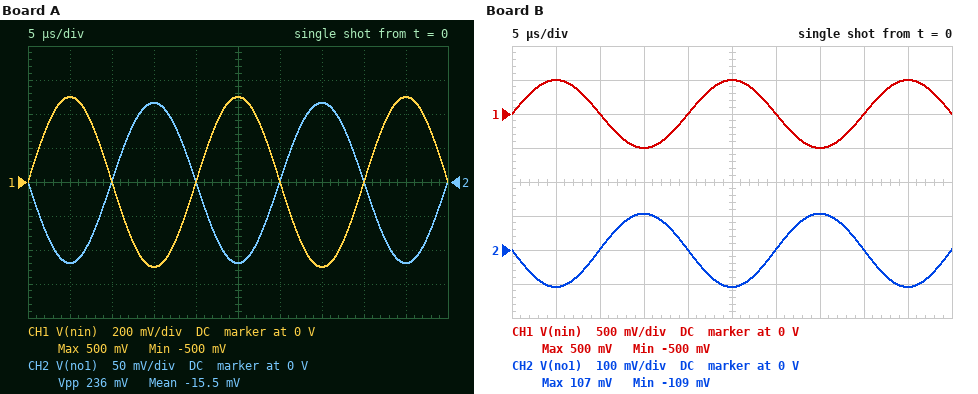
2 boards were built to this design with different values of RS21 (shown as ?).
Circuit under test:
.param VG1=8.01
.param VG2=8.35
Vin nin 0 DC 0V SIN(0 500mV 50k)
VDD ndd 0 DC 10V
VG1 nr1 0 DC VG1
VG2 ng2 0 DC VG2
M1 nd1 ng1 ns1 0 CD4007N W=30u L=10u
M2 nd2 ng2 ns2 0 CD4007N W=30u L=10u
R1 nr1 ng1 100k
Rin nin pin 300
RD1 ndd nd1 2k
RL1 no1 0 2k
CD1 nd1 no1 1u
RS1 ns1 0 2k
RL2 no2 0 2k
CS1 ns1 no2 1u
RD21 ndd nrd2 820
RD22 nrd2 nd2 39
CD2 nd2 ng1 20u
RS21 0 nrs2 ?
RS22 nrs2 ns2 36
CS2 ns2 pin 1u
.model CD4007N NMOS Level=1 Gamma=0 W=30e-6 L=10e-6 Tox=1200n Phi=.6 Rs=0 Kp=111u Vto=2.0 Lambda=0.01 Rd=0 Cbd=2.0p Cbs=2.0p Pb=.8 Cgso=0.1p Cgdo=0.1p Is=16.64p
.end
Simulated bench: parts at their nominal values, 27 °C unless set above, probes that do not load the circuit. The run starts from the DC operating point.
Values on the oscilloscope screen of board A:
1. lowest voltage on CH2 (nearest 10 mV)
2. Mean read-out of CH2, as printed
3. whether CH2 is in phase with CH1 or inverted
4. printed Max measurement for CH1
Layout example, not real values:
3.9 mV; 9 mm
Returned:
-120 mV; -15.5 mV; inverted; 500 mV
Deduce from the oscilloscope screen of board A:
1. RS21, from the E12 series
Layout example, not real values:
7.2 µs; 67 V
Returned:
180 Ω
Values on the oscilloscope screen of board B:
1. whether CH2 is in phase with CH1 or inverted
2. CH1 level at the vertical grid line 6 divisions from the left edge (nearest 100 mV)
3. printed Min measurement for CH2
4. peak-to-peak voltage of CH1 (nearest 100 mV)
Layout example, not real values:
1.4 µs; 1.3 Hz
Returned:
inverted; 0 V; -109 mV; 1.0 V
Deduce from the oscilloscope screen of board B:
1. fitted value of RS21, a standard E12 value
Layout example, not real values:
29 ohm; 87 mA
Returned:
150 Ω
